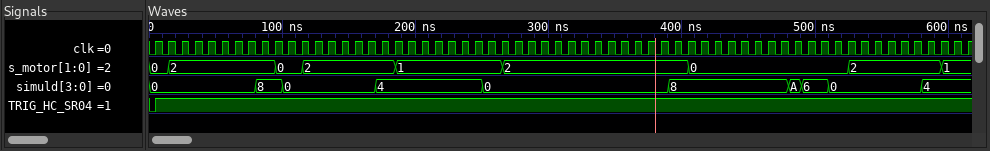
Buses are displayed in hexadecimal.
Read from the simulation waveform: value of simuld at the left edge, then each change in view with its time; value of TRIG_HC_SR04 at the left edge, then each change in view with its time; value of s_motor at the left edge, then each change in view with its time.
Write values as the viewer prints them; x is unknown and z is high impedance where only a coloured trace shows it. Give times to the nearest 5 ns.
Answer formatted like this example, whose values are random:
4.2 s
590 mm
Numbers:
0, 8 at 80 ns, 0 at 100 ns, 4 at 170 ns, 0 at 250 ns, 8 at 390 ns, A at 480 ns, 6 at 490 ns, 0 at 510 ns, 4 at 580 ns
0, 1 at 5 ns
0, 2 at 15 ns, 0 at 95 ns, 2 at 115 ns, 1 at 185 ns, 2 at 265 ns, 0 at 405 ns, 2 at 525 ns, 1 at 595 ns
